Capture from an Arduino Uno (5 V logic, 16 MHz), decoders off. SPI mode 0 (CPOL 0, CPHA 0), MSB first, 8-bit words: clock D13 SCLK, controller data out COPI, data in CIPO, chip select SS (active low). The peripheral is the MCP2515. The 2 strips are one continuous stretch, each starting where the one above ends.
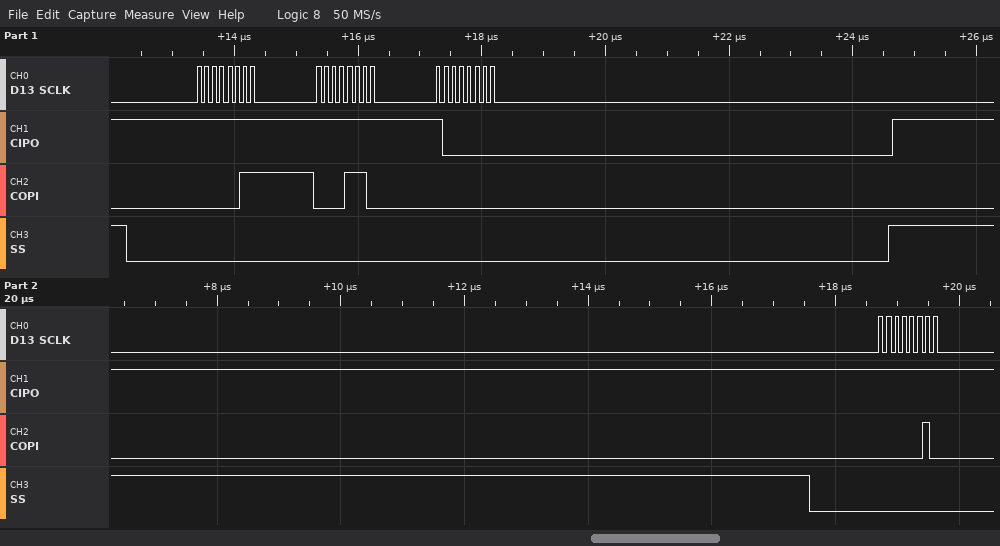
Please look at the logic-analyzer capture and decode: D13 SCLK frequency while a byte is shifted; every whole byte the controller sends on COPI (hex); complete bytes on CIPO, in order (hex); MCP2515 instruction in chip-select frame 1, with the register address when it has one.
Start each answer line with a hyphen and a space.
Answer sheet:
- 8 MHz
- 03 0E 00 02
- FF FF 80 FF
- READ 0x0E
